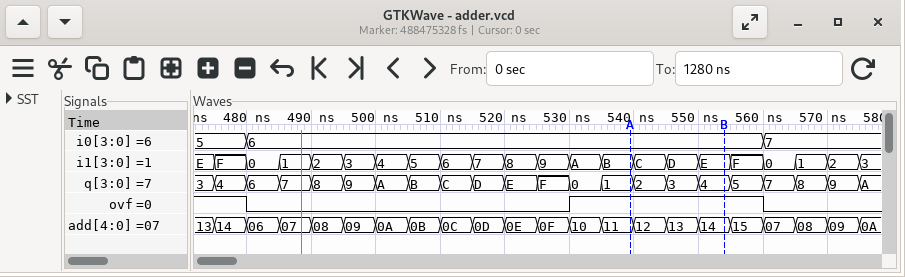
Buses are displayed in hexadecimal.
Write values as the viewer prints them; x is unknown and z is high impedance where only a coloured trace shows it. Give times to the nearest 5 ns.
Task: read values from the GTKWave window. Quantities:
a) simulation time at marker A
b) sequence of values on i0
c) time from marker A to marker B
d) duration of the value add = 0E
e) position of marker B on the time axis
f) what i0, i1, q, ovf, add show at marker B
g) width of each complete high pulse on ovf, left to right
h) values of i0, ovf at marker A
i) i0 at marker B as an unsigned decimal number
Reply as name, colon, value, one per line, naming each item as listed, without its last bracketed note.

simulation time at marker A: 540 ns
sequence of values on i0: 5, 6, 7
time from marker A to marker B: 15 ns
duration of the value add = 0E: 5 ns
position of marker B on the time axis: 555 ns
what i0, i1, q, ovf, add show at marker B: i0=6, i1=E, q=4, ovf=1, add=14
width of each complete high pulse on ovf, left to right: 30 ns
values of i0, ovf at marker A: i0=6, ovf=1
i0 at marker B as an unsigned decimal number: 6
